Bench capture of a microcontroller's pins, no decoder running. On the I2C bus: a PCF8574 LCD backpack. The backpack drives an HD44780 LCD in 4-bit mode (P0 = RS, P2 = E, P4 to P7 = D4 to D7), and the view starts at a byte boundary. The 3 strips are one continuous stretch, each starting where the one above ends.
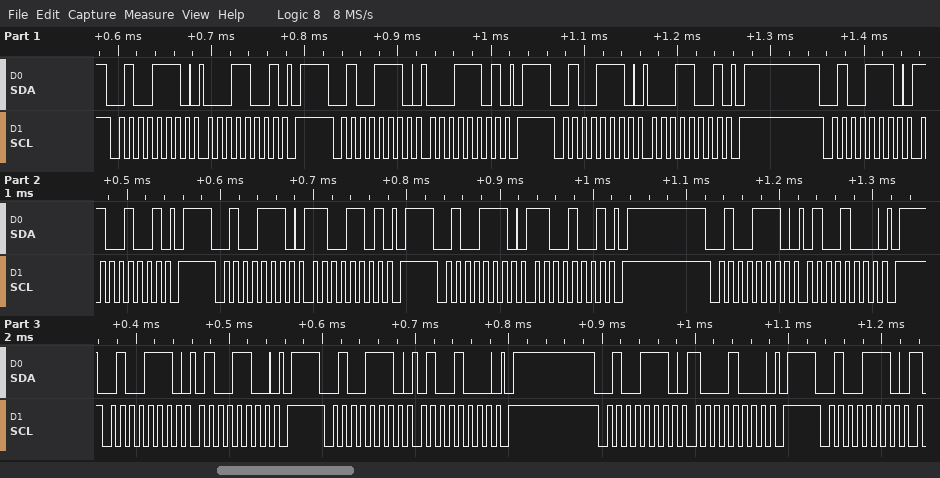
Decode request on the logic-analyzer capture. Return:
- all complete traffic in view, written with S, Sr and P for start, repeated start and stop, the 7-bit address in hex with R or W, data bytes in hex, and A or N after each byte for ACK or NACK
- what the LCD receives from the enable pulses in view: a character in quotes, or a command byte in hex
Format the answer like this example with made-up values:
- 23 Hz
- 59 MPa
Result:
- S 27W A 19 A P S 27W A 1D A P S 27W A 19 A P S 27W A C9 A P S 27W A CD A P S 27W A C9 A P S 27W A 48 A P S 27W A 4C A P S 27W A 48 A P S 27W A 88 A P S 27W A
- data 0x1C
